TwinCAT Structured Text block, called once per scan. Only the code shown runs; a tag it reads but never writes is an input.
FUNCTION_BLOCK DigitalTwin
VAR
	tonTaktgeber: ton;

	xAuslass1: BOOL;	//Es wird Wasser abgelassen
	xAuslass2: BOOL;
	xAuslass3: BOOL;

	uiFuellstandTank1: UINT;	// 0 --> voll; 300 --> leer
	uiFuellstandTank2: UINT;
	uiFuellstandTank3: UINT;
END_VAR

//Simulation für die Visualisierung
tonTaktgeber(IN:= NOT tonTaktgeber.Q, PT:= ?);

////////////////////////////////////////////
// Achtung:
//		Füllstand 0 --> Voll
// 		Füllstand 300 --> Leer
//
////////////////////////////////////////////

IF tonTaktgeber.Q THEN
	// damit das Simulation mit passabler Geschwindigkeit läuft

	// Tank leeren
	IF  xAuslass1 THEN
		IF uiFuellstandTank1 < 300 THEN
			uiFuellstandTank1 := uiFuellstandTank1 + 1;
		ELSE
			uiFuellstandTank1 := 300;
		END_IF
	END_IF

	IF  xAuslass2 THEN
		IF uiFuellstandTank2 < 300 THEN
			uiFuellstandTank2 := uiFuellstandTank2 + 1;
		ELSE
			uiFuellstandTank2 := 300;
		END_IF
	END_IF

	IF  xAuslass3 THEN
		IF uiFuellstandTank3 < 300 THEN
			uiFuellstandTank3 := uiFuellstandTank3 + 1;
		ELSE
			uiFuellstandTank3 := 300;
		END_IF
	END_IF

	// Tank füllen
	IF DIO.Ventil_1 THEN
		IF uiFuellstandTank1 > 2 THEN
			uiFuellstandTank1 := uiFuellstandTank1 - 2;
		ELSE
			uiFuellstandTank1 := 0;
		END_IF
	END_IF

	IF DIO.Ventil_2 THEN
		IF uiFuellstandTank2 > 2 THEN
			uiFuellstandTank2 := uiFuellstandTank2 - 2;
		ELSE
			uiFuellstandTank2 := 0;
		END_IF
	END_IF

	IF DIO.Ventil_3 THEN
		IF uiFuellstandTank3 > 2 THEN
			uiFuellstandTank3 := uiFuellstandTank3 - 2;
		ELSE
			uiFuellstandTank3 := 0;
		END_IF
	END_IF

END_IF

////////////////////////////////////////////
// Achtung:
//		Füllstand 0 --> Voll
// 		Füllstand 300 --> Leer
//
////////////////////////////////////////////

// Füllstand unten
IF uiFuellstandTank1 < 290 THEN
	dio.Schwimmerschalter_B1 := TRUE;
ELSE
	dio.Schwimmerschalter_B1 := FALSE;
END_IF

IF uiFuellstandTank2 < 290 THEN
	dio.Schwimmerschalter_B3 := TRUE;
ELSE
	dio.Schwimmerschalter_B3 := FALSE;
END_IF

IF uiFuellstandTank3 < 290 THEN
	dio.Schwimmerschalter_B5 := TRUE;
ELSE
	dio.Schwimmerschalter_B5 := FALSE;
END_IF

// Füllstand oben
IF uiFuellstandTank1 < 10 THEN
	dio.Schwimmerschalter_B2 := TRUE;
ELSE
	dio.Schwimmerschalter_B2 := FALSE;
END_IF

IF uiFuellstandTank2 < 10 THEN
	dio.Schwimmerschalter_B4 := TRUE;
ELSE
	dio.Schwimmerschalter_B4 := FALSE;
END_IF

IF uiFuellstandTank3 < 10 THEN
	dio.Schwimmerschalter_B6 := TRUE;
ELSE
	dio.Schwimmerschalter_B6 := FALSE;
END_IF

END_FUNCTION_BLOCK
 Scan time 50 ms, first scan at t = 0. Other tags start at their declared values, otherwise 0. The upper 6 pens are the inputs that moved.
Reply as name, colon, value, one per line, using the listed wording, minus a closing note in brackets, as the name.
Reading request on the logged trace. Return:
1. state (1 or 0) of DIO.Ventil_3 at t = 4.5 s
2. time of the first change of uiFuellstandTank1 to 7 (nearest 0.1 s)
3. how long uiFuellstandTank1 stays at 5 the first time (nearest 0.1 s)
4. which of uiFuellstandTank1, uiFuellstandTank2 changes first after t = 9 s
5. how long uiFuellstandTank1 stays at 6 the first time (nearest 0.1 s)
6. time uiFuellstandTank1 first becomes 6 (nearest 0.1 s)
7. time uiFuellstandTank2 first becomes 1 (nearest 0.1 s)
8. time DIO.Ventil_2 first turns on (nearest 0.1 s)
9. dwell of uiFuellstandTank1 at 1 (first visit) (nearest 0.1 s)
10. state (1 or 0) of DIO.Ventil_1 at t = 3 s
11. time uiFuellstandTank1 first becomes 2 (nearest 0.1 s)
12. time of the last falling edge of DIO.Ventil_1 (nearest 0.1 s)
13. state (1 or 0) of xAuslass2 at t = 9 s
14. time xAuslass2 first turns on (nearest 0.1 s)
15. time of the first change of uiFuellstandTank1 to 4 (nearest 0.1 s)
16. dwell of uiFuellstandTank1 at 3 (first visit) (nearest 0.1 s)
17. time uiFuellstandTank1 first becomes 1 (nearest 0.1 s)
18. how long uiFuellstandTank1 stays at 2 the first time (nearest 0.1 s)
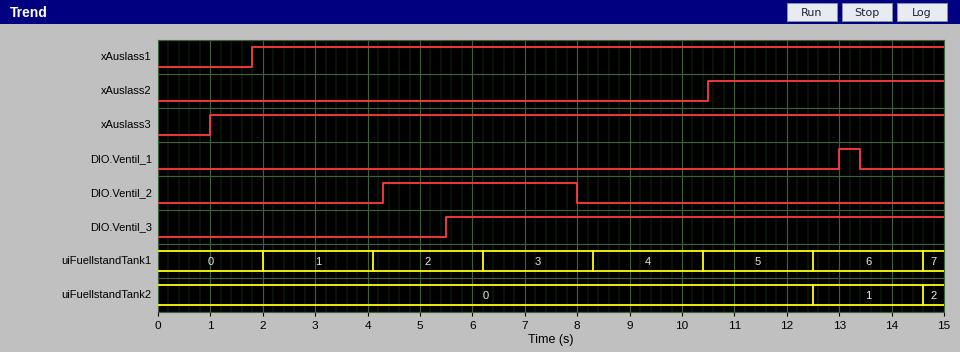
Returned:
state (1 or 0) of DIO.Ventil_3 at t = 4.5 s: 0
time of the first change of uiFuellstandTank1 to 7: 14.6 s
how long uiFuellstandTank1 stays at 5 the first time: 2.1 s
which of uiFuellstandTank1, uiFuellstandTank2 changes first after t = 9 s: uiFuellstandTank1
how long uiFuellstandTank1 stays at 6 the first time: 2.1 s
time uiFuellstandTank1 first becomes 6: 12.5 s
time uiFuellstandTank2 first becomes 1: 12.5 s
time DIO.Ventil_2 first turns on: 4.3 s
dwell of uiFuellstandTank1 at 1 (first visit): 2.1 s
state (1 or 0) of DIO.Ventil_1 at t = 3 s: 0
time uiFuellstandTank1 first becomes 2: 4.1 s
time of the last falling edge of DIO.Ventil_1: 13.4 s
state (1 or 0) of xAuslass2 at t = 9 s: 0
time xAuslass2 first turns on: 10.5 s
time of the first change of uiFuellstandTank1 to 4: 8.3 s
dwell of uiFuellstandTank1 at 3 (first visit): 2.1 s
time uiFuellstandTank1 first becomes 1: 2.0 s
how long uiFuellstandTank1 stays at 2 the first time: 2.1 s
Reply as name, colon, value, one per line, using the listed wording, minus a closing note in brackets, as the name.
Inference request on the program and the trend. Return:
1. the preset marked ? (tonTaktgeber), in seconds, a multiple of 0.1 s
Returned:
the preset marked ? (tonTaktgeber), in seconds, a multiple of 0.1 s: 2.0 s
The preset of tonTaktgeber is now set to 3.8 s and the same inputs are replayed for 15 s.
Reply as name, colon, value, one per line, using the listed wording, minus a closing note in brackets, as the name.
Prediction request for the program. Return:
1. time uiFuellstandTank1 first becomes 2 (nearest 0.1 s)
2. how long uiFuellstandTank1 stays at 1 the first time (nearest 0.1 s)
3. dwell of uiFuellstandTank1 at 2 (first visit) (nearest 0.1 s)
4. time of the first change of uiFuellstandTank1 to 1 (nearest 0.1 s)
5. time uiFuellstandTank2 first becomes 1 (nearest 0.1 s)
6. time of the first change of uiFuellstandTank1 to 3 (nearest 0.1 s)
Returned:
time uiFuellstandTank1 first becomes 2: 7.7 s
how long uiFuellstandTank1 stays at 1 the first time: 3.9 s
dwell of uiFuellstandTank1 at 2 (first visit): 3.9 s
time of the first change of uiFuellstandTank1 to 1: 3.8 s
time uiFuellstandTank2 first becomes 1: 11.6 s
time of the first change of uiFuellstandTank1 to 3: 11.6 s
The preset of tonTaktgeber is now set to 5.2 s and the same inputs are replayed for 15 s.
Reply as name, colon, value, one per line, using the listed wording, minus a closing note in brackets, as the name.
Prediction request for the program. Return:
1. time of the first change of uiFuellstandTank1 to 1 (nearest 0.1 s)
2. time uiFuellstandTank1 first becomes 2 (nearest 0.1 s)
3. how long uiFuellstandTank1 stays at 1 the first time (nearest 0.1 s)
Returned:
time of the first change of uiFuellstandTank1 to 1: 5.2 s
time uiFuellstandTank1 first becomes 2: 10.5 s
how long uiFuellstandTank1 stays at 1 the first time: 5.3 s
